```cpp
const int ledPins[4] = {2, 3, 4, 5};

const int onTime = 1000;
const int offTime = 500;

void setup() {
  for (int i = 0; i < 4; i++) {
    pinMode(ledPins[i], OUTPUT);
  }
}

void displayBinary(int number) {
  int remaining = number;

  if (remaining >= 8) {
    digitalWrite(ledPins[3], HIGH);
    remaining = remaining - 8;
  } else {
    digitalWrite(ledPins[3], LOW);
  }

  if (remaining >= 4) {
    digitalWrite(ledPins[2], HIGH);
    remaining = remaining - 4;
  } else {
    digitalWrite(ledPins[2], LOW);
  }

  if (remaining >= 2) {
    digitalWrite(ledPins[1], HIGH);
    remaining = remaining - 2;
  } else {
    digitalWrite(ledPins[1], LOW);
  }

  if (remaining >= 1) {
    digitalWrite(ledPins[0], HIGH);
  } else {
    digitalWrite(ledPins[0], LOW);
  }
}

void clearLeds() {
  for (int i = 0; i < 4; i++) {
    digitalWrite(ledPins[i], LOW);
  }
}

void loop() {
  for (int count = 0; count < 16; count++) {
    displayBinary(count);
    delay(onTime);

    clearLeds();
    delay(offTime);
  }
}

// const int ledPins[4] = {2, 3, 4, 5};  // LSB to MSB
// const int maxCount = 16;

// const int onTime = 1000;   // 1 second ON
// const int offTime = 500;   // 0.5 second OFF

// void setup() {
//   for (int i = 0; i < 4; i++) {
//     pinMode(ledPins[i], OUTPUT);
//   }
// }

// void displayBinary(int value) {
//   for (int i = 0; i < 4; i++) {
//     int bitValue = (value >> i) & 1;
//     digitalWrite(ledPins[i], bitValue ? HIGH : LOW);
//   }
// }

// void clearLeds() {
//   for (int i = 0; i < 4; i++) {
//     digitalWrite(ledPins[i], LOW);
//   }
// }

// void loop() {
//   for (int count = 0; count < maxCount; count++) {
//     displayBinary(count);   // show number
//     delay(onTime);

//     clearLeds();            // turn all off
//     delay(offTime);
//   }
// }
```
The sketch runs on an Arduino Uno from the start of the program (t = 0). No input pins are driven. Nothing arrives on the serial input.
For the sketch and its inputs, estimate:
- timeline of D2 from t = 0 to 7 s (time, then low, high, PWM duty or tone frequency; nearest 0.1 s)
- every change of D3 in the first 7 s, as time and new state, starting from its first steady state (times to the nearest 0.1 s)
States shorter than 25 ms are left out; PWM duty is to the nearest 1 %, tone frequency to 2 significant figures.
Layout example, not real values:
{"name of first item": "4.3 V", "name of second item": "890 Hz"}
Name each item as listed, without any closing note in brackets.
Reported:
{"timeline of D2 from t = 0 to 7 s": "0 s low; 1.5 s high; 2.5 s low; 4.5 s high; 5.5 s low", "every change of D3 in the first 7 s, as time and new state, starting from its first steady state": "0 s low; 3 s high; 4 s low; 4.5 s high; 5.5 s low"}
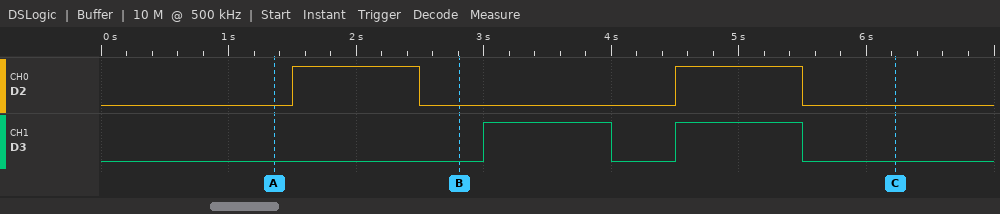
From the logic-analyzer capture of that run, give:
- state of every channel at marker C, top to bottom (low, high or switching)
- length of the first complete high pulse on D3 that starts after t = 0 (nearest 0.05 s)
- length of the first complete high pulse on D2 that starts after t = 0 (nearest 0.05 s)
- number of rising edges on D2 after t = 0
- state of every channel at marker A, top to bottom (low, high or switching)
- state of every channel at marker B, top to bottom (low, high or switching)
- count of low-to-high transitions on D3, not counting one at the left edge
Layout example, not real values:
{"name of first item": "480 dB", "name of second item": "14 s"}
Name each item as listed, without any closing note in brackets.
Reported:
{"state of every channel at marker C, top to bottom": "D2 low, D3 low", "length of the first complete high pulse on D3 that starts after t = 0": "1.00 s", "length of the first complete high pulse on D2 that starts after t = 0": "1.00 s", "number of rising edges on D2 after t = 0": "2", "state of every channel at marker A, top to bottom": "D2 low, D3 low", "state of every channel at marker B, top to bottom": "D2 low, D3 low", "count of low-to-high transitions on D3, not counting one at the left edge": "2"}
